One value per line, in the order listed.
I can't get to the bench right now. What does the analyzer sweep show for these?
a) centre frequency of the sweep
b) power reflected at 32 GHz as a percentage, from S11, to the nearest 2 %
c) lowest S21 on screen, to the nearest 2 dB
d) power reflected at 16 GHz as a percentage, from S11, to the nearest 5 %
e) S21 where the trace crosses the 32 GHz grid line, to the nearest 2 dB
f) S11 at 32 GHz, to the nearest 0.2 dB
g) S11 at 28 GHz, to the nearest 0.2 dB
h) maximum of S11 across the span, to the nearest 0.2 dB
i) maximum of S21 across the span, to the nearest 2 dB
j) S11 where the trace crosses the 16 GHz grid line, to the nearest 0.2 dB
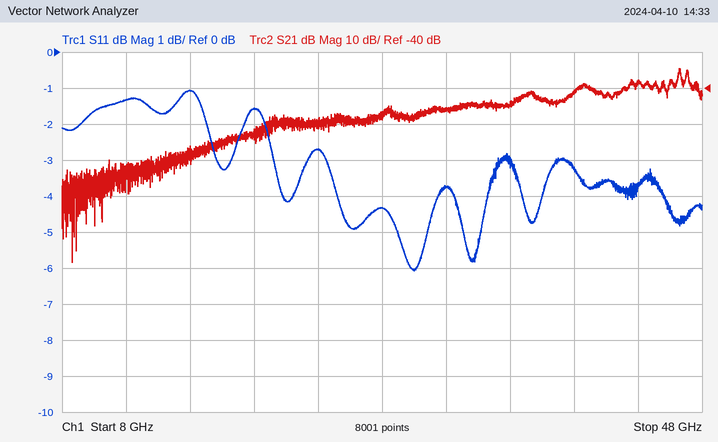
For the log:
28 GHz
42 %
-88 dB
80 %
-46 dB
-3.8 dB
-4.4 dB
-1.0 dB
-34 dB
-1.0 dB
